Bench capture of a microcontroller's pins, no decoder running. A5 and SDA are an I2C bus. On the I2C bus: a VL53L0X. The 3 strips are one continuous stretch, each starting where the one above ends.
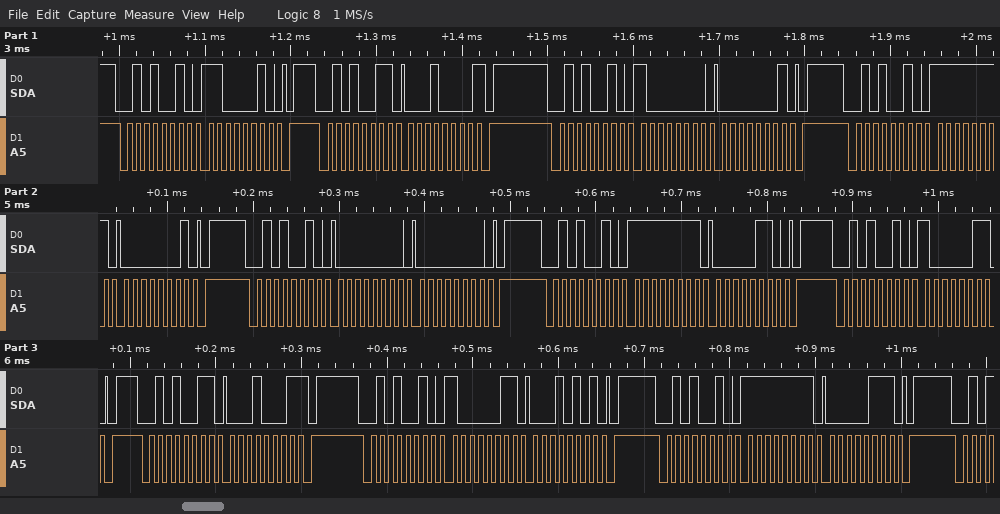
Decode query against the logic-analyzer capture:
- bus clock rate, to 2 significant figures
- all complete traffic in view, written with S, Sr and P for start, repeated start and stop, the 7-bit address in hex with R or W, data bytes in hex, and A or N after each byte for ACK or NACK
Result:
100 kHz
S 29W A C2 A P S 29R A 10 N P S 29W A 80 A 01 A P S 29W A FF A 01 A P S 29W A 00 A 00 A P S 29W A FF A 06 A P S 29W A 83 A P S 29R A 11 N P S 29W A 83 A 15 A P S 29W A FF A 07 A P
